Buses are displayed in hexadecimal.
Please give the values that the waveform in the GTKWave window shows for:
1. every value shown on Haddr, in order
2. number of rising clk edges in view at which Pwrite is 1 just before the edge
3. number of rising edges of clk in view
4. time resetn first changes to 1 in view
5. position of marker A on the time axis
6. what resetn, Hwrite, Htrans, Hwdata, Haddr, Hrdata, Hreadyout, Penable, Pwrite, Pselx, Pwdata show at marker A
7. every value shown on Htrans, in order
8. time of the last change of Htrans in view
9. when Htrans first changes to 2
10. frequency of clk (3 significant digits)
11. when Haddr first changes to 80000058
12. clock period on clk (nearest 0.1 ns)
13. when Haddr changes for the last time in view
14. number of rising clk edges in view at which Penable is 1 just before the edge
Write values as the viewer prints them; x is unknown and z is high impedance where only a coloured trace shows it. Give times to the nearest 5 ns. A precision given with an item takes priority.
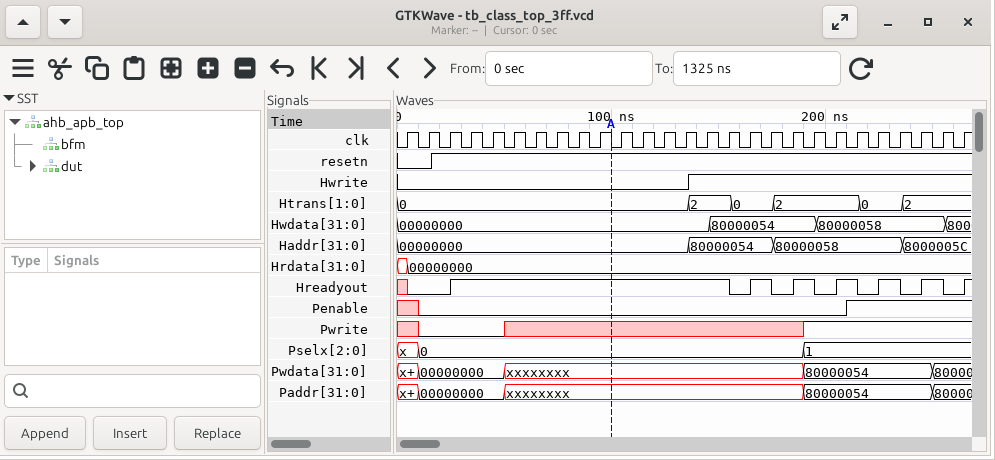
00000000, 80000054, 80000058, 8000005C
8
27
15 ns
100 ns
resetn=1, Hwrite=0, Htrans=0, Hwdata=00000000, Haddr=00000000, Hrdata=00000000, Hreadyout=1, Penable=0, Pwrite=x, Pselx=0, Pwdata=xxxxxxxx
0, 2, 0, 2, 0, 2
235 ns
135 ns
100 MHz
175 ns
10 ns
235 ns
6
